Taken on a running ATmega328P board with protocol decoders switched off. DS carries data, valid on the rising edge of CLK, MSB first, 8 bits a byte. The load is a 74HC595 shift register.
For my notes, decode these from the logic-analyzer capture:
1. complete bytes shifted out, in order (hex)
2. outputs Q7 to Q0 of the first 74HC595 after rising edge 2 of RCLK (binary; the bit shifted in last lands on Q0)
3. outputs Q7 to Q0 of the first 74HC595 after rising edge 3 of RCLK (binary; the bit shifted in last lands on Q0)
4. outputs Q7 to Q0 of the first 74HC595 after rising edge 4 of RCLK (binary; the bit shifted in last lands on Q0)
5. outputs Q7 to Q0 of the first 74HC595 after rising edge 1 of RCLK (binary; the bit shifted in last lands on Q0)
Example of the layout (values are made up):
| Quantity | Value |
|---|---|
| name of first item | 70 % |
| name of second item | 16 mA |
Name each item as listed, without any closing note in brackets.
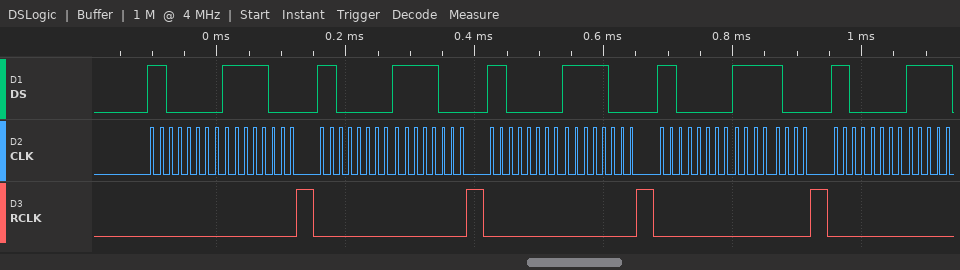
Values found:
| Quantity | Value |
|---|---|
| complete bytes shifted out, in order | C0 F8 C0 F8 C0 F8 C0 F8 C0 |
| outputs Q7 to Q0 of the first 74HC595 after rising edge 2 of RCLK | 11111000 |
| outputs Q7 to Q0 of the first 74HC595 after rising edge 3 of RCLK | 11111000 |
| outputs Q7 to Q0 of the first 74HC595 after rising edge 4 of RCLK | 11111000 |
| outputs Q7 to Q0 of the first 74HC595 after rising edge 1 of RCLK | 11111000 |
